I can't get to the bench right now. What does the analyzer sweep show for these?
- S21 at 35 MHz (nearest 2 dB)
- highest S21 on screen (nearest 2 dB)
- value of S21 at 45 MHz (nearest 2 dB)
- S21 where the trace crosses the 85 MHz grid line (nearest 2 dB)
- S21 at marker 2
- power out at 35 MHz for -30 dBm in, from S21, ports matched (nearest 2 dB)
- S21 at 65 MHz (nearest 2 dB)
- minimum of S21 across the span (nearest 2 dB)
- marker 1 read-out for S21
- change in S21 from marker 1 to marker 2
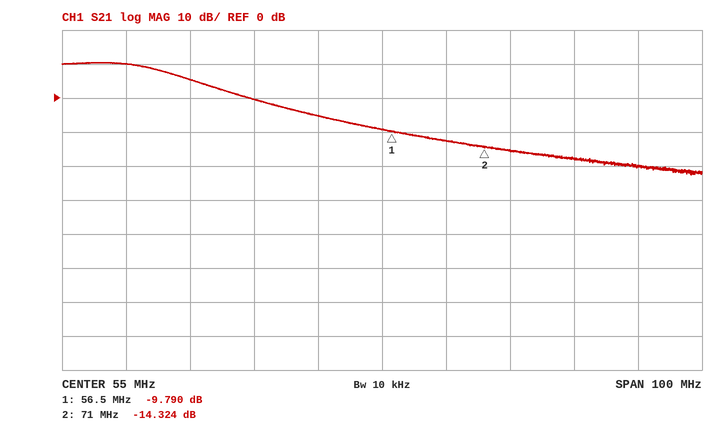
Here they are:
0 dB
10 dB
-6 dB
-18 dB
-14.324 dB
-30 dBm
-12 dB
-22 dB
-9.790 dB
-4.534 dB
